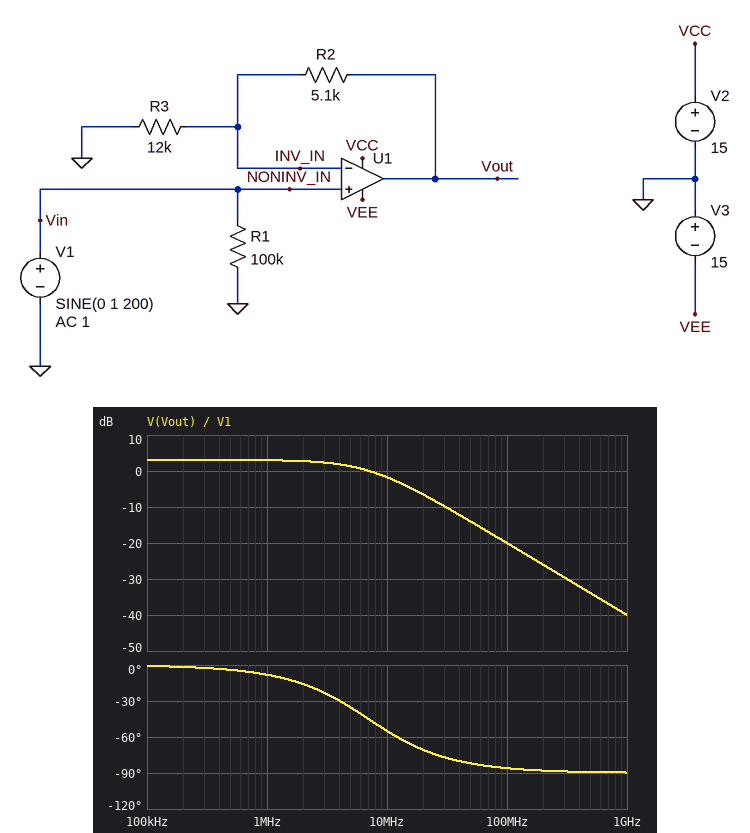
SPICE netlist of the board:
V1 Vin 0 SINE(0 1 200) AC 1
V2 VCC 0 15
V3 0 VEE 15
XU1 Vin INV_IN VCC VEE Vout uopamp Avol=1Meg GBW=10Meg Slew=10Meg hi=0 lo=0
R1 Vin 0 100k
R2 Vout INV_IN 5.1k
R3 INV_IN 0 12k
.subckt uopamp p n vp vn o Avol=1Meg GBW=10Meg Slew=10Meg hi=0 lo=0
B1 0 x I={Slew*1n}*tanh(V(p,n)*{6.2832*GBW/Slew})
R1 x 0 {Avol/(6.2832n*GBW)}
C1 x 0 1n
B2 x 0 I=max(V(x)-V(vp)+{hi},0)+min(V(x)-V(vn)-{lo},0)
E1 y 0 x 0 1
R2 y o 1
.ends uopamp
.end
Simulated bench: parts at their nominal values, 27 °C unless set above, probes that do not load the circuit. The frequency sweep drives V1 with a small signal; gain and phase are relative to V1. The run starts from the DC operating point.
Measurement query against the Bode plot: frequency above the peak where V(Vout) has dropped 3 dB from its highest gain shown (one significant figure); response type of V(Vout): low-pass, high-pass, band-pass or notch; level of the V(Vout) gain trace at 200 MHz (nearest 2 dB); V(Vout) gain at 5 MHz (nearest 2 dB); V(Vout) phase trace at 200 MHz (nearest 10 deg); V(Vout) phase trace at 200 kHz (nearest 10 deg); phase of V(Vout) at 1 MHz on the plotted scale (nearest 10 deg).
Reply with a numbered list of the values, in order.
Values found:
1. 7 MHz
2. low-pass
3. -26 dB
4. 2 dB
5. -90 deg
6. 0 deg
7. -10 deg
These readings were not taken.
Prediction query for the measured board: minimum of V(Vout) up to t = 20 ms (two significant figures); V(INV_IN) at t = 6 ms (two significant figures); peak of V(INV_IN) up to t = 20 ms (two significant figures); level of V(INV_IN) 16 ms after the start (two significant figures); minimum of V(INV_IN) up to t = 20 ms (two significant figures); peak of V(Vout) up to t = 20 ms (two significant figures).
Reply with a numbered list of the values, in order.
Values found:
1. -1.4 V
2. 950 mV
3. 1.0 V
4. 950 mV
5. -1.0 V
6. 1.4 V
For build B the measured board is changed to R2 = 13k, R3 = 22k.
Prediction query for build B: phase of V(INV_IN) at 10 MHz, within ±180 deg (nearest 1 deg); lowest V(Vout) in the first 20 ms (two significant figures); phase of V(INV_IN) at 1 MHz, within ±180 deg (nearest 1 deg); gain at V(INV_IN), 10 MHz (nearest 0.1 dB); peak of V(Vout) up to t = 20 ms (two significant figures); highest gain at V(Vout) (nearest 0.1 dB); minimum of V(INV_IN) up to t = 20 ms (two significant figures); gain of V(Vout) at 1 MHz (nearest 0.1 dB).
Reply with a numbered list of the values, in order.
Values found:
1. -58 deg
2. -1.6 V
3. -9 deg
4. -5.5 dB
5. 1.6 V
6. 4.0 dB
7. -1.0 V
8. 3.9 dB
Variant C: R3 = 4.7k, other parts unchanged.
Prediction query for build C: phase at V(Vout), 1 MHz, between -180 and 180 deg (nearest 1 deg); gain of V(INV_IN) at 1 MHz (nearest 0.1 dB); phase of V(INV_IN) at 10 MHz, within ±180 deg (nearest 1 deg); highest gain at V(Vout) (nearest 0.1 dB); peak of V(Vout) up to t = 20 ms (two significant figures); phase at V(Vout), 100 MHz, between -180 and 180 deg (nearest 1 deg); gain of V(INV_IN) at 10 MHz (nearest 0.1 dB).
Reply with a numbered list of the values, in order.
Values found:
1. -12 deg
2. -0.2 dB
3. -64 deg
4. 6.4 dB
5. 2.1 V
6. -87 deg
7. -7.3 dB
